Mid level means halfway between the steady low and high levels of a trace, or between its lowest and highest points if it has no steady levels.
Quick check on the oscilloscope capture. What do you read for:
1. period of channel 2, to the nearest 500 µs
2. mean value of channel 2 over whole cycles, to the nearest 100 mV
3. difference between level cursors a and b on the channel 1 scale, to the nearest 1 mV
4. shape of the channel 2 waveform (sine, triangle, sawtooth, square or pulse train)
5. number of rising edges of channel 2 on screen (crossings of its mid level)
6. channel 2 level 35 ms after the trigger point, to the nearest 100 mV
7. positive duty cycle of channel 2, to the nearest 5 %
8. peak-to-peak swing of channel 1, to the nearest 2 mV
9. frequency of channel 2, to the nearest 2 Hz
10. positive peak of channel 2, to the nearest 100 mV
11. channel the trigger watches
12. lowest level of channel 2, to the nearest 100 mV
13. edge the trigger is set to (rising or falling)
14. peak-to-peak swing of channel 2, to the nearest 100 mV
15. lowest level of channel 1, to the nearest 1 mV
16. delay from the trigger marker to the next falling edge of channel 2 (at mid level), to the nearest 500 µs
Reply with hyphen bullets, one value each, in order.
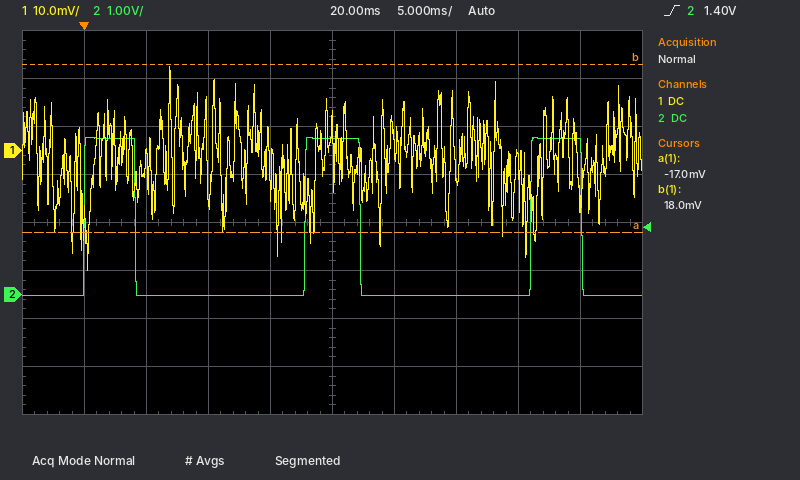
- 18.0 ms
- 800 mV
- 35 mV
- pulse train
- 3
- 0.0 V
- 25 %
- 42 mV
- 56 Hz
- 3.3 V
- channel 2
- 0.0 V
- rising
- 3.3 V
- -25 mV
- 4.0 ms
